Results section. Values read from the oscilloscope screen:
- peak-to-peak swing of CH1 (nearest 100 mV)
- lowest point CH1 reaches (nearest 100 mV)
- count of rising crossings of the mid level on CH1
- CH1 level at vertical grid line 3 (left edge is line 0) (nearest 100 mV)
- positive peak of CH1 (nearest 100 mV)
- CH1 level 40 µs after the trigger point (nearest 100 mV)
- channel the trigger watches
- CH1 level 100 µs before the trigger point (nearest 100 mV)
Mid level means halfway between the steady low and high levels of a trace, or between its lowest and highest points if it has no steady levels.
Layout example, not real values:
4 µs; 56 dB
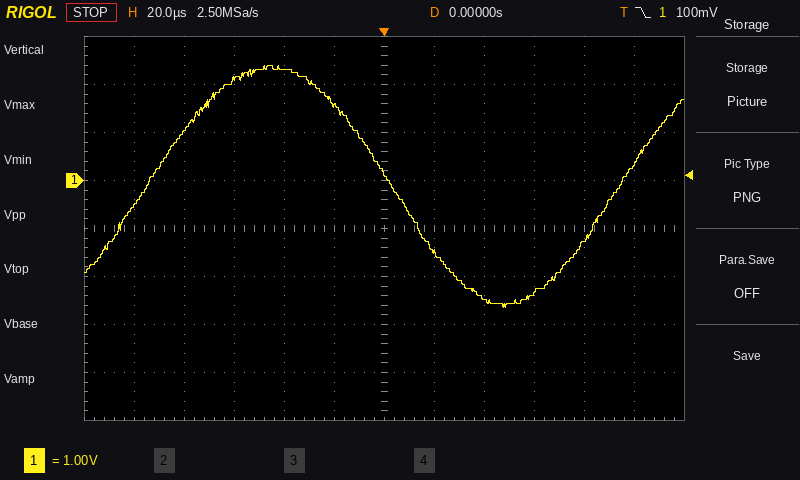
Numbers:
5.0 V; -2.6 V; 2; 2.1 V; 2.4 V; -2.5 V; CH1; -500 mV
